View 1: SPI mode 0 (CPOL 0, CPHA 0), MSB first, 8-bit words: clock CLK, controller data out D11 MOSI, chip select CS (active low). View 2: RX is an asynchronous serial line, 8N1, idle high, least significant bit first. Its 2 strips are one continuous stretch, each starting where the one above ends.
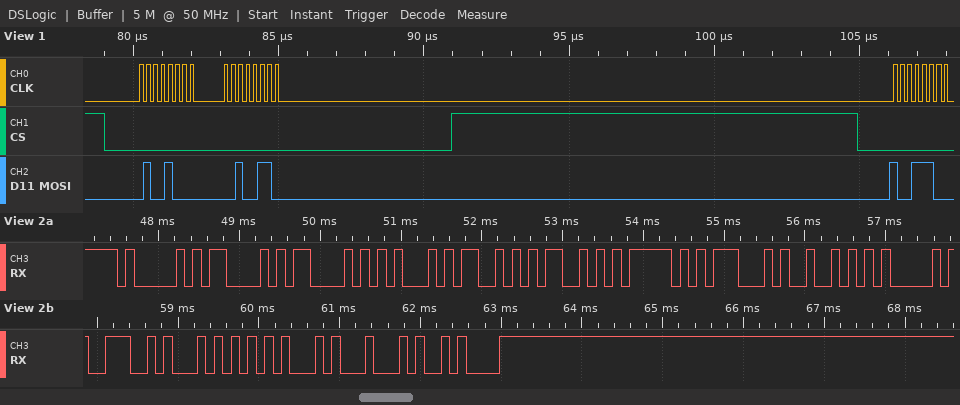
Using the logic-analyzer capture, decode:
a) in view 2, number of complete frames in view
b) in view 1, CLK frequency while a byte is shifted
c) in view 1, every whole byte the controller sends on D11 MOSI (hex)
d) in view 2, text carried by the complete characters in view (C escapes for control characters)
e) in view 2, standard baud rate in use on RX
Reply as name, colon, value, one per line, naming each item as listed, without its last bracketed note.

in view 2, number of complete frames in view: 15
in view 1, CLK frequency while a byte is shifted: 4 MHz
in view 1, every whole byte the controller sends on D11 MOSI: 48 26 9C
in view 2, text carried by the complete characters in view: "ACCESS_GRANTED\n"
in view 2, standard baud rate in use on RX: 9600 baud
